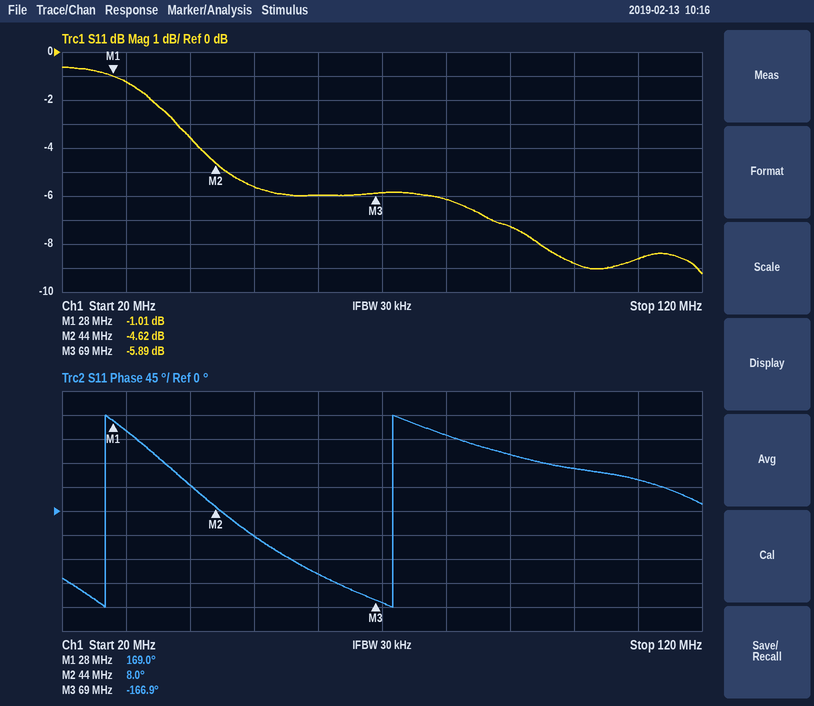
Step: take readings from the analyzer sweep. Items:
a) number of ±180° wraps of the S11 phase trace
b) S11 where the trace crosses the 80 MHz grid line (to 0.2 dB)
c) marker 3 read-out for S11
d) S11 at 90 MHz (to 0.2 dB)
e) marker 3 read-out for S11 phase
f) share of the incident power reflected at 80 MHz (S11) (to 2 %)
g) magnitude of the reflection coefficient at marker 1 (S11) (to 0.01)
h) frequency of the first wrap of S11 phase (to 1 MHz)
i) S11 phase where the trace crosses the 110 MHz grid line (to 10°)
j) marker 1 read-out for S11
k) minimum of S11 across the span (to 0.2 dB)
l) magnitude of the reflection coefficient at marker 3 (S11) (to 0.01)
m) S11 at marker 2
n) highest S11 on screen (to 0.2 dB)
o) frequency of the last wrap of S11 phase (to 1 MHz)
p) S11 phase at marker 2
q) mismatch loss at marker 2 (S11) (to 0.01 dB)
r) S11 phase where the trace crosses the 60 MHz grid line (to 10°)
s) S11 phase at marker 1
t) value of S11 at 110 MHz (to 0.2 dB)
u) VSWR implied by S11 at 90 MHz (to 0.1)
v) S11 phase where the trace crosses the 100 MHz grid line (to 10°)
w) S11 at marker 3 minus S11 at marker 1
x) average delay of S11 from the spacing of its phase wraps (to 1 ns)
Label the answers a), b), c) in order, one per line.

a) 2
b) -6.2 dB
c) -5.89 dB
d) -7.2 dB
e) -166.9°
f) 24 %
g) 0.89
h) 27 MHz
i) 60°
j) -1.01 dB
k) -9.2 dB
l) 0.51
m) -4.62 dB
n) -0.6 dB
o) 72 MHz
p) 8.0°
q) 1.84 dB
r) -120°
s) 169.0°
t) -8.6 dB
u) 2.5
v) 80°
w) -4.88 dB
x) 22 ns
